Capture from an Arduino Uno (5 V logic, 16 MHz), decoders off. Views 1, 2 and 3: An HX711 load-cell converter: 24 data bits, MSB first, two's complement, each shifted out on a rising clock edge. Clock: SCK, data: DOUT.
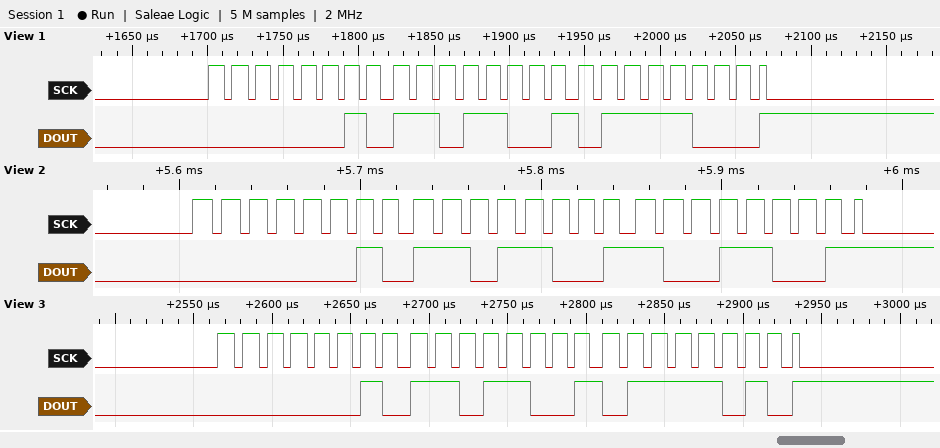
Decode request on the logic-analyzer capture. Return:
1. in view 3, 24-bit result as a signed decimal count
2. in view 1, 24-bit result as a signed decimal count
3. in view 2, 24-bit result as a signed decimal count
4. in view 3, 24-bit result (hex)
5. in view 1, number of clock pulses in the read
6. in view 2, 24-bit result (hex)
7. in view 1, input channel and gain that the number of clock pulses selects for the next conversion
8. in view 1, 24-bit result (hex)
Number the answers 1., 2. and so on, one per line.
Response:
1. 186746
2. 186744
3. 186777
4. 0x02D97A
5. 25
6. 0x02D999
7. channel A, gain 128
8. 0x02D978
